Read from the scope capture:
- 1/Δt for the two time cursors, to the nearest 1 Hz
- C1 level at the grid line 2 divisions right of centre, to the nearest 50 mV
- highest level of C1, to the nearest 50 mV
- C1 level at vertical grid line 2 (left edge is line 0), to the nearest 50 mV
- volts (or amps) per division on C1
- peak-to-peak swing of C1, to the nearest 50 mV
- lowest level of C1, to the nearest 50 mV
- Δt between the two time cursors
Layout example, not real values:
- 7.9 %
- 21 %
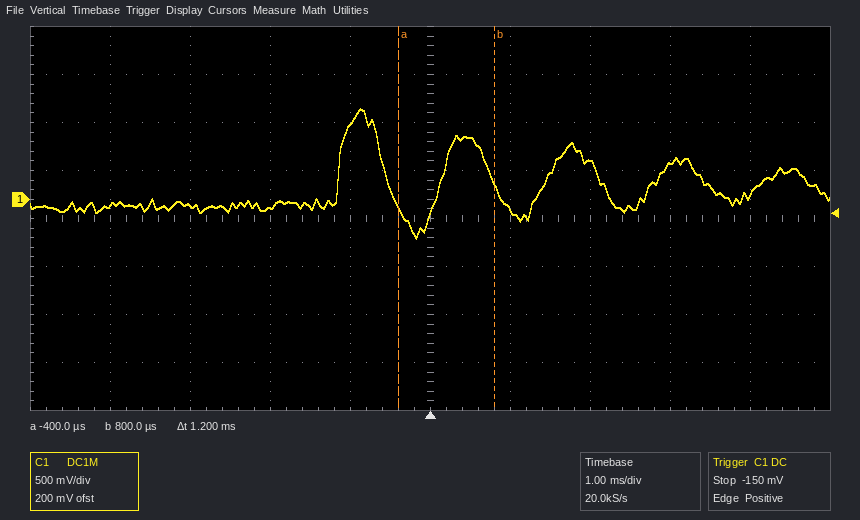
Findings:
- 833 Hz
- 400 mV
- 950 mV
- -50 mV
- 500 mV
- 1.35 V
- -400 mV
- 1.2 ms
